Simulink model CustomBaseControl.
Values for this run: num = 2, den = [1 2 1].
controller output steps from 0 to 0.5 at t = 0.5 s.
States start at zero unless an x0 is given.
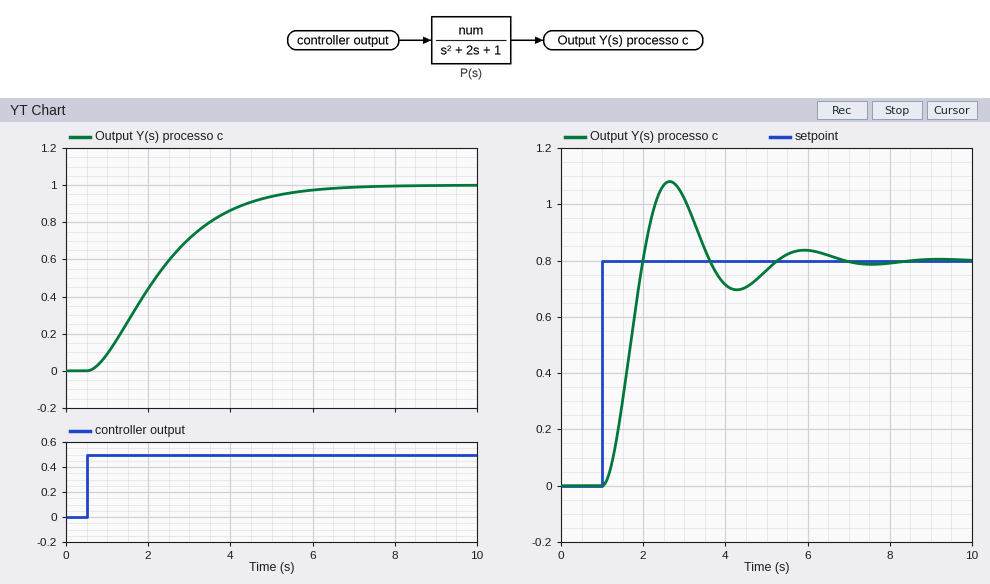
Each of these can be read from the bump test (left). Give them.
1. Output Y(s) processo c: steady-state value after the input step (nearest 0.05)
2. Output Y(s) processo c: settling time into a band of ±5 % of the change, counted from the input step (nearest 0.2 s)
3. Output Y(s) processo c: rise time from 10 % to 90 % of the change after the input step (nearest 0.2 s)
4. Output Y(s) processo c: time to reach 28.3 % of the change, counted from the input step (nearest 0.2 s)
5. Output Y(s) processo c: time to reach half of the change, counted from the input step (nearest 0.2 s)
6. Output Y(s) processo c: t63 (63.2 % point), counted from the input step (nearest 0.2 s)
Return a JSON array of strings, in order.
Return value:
["1.00", "4.8 s", "3.4 s", "1.0 s", "1.6 s", "2.2 s"]
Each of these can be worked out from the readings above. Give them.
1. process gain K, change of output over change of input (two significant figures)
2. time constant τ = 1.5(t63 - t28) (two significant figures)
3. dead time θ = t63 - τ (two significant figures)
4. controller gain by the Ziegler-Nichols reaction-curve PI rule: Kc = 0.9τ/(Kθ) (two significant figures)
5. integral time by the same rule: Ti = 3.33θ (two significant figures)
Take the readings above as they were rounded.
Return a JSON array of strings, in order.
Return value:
["2.0", "1.8 s", "0.40 s", "2.0", "1.3 s"]
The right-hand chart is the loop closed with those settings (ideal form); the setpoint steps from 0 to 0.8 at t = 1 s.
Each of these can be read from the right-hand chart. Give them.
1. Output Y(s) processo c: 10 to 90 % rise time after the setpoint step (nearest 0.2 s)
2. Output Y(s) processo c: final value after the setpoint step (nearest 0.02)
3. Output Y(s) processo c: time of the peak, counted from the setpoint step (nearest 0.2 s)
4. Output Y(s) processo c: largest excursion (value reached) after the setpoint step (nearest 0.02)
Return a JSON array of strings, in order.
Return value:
["0.6 s", "0.80", "1.6 s", "1.08"]
